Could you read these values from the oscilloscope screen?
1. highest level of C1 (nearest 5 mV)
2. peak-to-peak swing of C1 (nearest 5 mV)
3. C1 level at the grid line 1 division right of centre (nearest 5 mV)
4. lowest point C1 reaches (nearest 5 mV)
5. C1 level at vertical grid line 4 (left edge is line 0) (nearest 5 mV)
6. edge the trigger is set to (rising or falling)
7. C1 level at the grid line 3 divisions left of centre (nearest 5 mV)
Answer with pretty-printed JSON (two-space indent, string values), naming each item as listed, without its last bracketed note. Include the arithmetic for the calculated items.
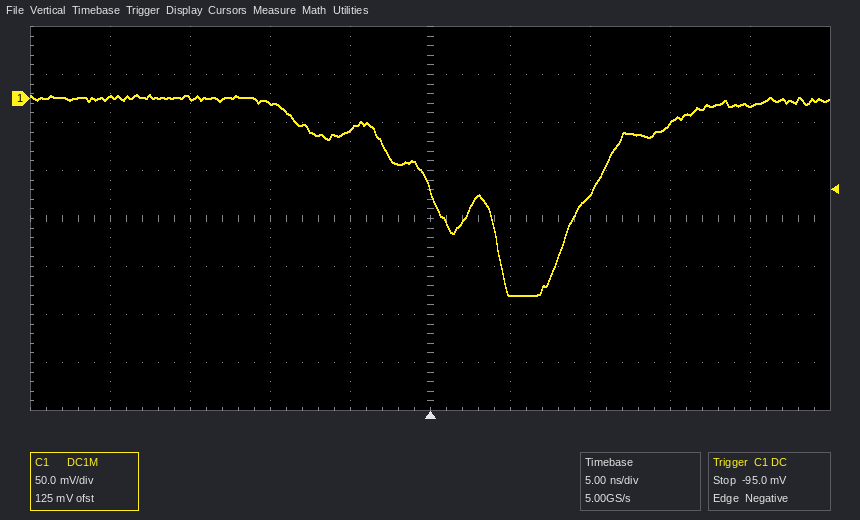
{
  "highest level of C1": "5 mV",
  "peak-to-peak swing of C1": "5 mV − (-205 mV) = 210 mV",
  "C1 level at the grid line 1 division right of centre": "-200 mV",
  "lowest point C1 reaches": "-205 mV",
  "C1 level at vertical grid line 4 (left edge is line 0)": "-30 mV",
  "edge the trigger is set to": "falling",
  "C1 level at the grid line 3 divisions left of centre": "0 mV"
}
